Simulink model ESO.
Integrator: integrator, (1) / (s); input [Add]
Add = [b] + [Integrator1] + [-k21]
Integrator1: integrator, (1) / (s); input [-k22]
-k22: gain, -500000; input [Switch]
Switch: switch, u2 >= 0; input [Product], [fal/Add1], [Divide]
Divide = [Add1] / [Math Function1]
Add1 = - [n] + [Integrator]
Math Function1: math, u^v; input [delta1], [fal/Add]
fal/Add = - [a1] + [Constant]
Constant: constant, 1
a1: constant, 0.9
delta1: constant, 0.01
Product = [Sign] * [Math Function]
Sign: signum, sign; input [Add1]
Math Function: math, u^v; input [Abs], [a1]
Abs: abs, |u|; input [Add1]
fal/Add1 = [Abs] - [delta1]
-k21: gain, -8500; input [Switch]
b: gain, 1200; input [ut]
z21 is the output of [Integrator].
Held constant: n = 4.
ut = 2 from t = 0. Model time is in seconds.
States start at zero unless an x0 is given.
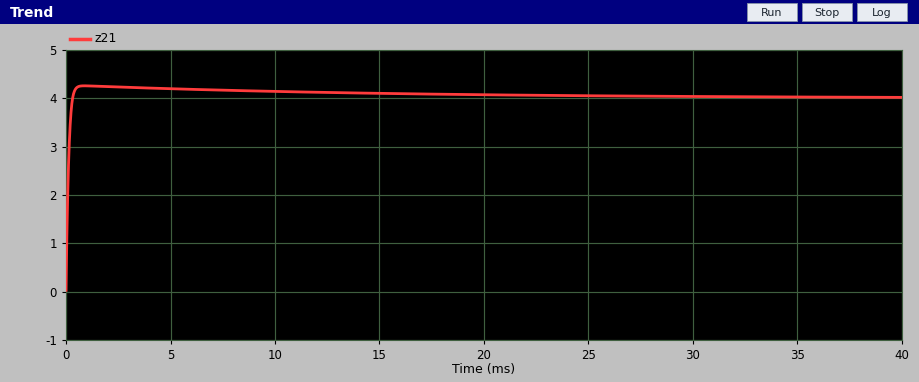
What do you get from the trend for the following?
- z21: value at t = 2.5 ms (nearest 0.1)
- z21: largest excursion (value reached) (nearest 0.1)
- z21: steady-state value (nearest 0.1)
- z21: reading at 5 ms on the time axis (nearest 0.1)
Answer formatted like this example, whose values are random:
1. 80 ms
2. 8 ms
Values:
1. 4.2
2. 4.3
3. 4.0
4. 4.2
